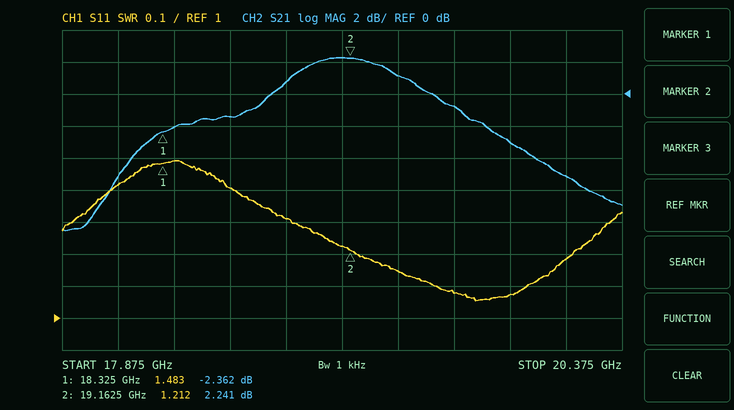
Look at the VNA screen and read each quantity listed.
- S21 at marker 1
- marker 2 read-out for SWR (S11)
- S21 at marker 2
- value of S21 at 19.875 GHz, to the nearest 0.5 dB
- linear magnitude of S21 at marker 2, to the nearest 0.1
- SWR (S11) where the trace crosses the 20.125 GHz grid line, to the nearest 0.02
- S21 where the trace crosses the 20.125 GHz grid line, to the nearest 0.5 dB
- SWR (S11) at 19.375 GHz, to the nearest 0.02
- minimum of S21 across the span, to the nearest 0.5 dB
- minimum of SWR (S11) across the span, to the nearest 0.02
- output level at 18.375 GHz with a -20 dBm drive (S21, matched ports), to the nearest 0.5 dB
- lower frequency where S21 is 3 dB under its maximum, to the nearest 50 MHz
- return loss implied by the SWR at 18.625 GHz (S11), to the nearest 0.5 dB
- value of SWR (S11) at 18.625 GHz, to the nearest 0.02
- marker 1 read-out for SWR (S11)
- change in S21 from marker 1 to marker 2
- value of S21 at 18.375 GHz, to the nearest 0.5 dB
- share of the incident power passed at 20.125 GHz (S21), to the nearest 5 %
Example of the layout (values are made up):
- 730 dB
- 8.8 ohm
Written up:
- -2.362 dB
- 1.212
- 2.241 dB
- -3.0 dB
- 1.3
- 1.18
- -5.0 dB
- 1.14
- -8.5 dB
- 1.06
- -22.0 dBm
- 18.75 GHz
- 15.5 dB
- 1.40
- 1.483
- 4.603 dB
- -2.0 dB
- 30 %
